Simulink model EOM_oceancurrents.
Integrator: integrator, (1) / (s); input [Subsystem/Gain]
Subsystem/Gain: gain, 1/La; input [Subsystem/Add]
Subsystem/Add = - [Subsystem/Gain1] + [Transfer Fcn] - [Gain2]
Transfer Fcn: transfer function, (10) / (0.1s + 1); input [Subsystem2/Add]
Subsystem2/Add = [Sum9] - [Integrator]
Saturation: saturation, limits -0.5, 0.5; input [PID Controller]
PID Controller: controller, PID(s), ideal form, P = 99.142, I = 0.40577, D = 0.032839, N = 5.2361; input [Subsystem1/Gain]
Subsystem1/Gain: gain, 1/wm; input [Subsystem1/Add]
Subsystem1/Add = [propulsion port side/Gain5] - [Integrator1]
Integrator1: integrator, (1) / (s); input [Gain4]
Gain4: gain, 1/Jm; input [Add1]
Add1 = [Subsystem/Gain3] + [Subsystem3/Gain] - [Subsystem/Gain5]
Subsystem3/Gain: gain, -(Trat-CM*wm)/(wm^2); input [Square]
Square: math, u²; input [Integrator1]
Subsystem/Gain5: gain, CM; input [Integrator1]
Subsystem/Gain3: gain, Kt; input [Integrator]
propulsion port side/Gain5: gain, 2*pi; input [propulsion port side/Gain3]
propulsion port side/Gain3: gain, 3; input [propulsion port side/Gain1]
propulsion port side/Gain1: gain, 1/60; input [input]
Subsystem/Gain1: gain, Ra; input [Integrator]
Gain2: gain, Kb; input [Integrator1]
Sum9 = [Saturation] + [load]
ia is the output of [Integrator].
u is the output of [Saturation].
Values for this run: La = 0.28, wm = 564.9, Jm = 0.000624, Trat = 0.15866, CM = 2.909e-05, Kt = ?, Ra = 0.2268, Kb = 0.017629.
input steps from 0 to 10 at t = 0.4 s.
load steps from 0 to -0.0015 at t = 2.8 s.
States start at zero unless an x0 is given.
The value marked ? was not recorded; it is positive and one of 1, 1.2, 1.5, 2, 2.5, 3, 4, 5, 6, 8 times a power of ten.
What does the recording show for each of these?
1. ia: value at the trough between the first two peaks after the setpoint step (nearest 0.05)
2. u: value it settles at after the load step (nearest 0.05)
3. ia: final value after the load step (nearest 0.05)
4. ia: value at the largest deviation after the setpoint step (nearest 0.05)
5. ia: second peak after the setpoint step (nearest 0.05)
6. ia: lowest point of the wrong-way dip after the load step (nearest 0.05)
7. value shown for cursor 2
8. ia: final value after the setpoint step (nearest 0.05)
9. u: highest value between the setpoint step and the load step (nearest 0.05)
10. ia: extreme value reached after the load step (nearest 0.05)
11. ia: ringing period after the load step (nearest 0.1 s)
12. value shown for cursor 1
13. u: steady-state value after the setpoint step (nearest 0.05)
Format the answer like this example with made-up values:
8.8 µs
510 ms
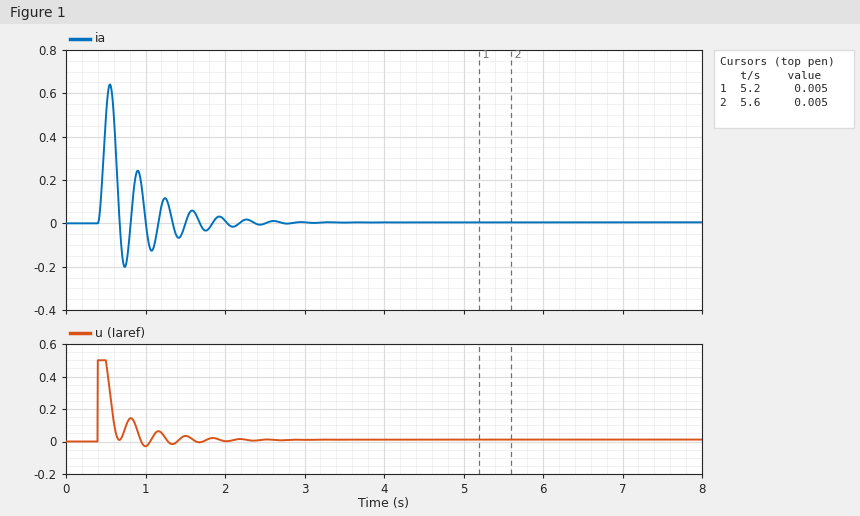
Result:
-0.20
0.00
0.00
0.65
0.25
0.00
0.005
0.00
0.50
0.00
0.3 s
0.005
0.00
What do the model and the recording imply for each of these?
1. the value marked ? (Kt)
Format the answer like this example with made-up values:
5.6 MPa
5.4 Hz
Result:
0.02
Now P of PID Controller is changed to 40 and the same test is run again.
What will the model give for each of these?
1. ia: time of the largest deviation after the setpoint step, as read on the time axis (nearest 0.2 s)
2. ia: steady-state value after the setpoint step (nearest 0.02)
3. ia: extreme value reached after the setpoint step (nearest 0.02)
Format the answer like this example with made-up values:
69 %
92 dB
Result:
0.6 s
0.00
0.32
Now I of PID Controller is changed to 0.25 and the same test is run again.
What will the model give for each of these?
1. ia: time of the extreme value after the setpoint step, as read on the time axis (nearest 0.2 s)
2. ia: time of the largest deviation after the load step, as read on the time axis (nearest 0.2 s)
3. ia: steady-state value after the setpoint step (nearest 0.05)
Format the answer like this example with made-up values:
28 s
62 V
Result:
0.6 s
3.0 s
0.00
